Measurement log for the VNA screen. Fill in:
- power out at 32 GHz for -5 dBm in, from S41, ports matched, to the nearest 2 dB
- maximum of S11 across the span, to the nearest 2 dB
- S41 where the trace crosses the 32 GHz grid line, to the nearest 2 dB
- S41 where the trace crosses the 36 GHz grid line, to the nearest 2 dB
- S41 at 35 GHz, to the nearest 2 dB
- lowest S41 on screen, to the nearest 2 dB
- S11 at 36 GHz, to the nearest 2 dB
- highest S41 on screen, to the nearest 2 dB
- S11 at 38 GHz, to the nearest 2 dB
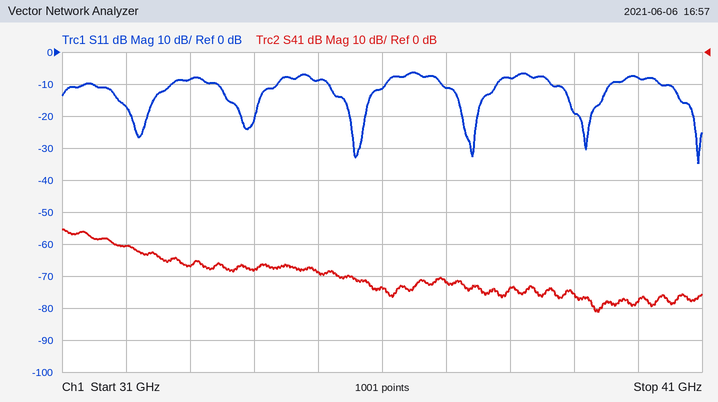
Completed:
-66 dBm
-6 dB
-60 dB
-74 dB
-68 dB
-82 dB
-12 dB
-56 dB
-8 dB
